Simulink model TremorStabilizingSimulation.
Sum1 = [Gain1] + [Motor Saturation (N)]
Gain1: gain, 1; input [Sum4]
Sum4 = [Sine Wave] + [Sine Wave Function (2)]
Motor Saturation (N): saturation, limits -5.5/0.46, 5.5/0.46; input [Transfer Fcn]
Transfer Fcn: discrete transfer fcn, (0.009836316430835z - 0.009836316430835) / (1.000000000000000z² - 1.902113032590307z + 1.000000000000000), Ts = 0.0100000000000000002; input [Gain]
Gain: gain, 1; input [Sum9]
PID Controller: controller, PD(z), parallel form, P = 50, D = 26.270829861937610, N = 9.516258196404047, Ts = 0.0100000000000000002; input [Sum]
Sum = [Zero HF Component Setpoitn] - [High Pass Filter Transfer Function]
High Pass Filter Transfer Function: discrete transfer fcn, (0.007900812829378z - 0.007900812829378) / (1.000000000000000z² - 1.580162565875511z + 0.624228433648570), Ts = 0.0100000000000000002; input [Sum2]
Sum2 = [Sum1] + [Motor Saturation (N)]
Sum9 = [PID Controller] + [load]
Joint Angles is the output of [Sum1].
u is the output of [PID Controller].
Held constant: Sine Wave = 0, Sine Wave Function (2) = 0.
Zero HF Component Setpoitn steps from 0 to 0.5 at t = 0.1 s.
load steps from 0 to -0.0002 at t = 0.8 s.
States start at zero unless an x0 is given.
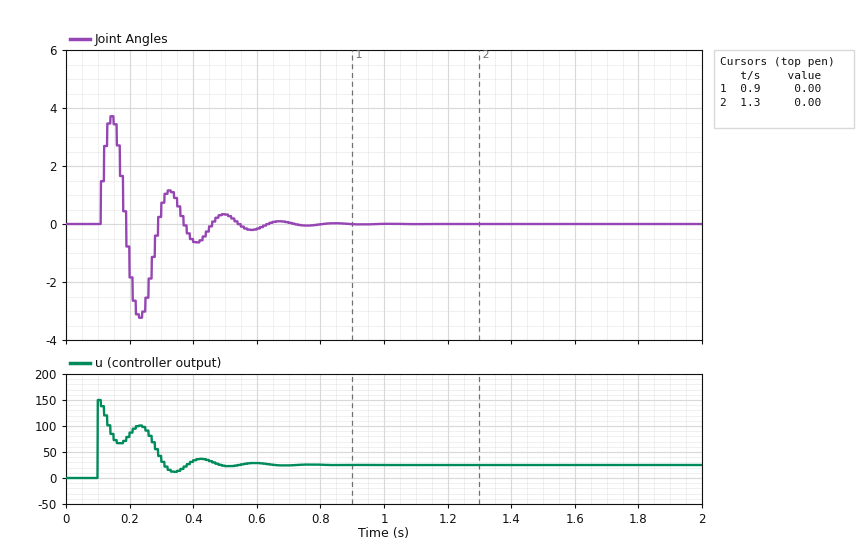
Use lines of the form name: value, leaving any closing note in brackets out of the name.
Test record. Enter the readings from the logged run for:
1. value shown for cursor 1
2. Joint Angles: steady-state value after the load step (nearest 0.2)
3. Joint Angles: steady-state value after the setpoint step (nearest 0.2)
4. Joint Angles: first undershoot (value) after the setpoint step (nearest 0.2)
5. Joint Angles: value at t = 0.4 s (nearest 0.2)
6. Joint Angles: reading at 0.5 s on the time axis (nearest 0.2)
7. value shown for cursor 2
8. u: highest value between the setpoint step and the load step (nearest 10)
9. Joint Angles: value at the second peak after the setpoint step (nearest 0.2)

value shown for cursor 1: 0.00
Joint Angles: steady-state value after the load step: 0.0
Joint Angles: steady-state value after the setpoint step: 0.0
Joint Angles: first undershoot (value) after the setpoint step: -3.2
Joint Angles: value at t = 0.4 s: -0.6
Joint Angles: reading at 0.5 s on the time axis: 0.4
value shown for cursor 2: 0.00
u: highest value between the setpoint step and the load step: 150
Joint Angles: value at the second peak after the setpoint step: 1.2
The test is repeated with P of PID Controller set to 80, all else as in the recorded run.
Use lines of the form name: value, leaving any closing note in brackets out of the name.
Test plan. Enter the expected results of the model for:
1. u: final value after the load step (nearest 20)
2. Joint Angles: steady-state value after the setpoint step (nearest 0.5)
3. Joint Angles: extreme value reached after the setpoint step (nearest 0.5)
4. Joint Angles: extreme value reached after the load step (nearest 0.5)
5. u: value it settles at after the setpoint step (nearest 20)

u: final value after the load step: 40
Joint Angles: steady-state value after the setpoint step: 0.0
Joint Angles: extreme value reached after the setpoint step: 4.0
Joint Angles: extreme value reached after the load step: 0.0
u: value it settles at after the setpoint step: 40
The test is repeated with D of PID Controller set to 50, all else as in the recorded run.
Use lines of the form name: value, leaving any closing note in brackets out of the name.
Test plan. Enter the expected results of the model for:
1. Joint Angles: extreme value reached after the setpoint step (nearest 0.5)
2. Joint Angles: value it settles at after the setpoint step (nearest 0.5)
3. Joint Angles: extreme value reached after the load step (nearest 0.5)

Joint Angles: extreme value reached after the setpoint step: 6.0
Joint Angles: value it settles at after the setpoint step: 0.0
Joint Angles: extreme value reached after the load step: 0.0
